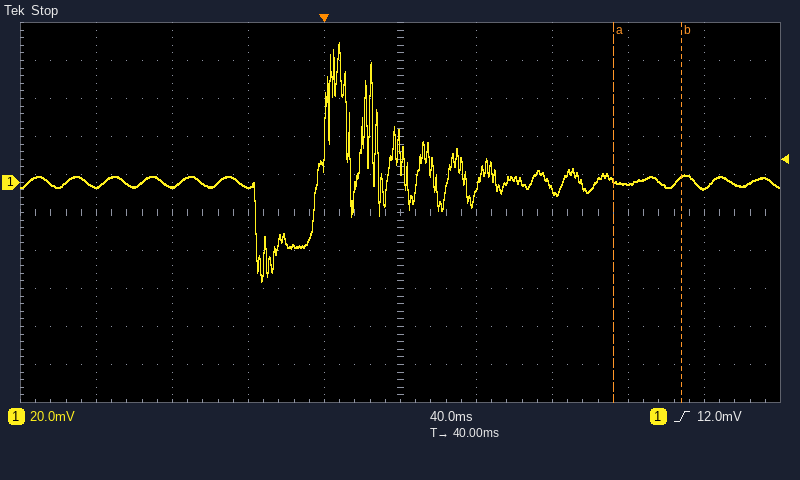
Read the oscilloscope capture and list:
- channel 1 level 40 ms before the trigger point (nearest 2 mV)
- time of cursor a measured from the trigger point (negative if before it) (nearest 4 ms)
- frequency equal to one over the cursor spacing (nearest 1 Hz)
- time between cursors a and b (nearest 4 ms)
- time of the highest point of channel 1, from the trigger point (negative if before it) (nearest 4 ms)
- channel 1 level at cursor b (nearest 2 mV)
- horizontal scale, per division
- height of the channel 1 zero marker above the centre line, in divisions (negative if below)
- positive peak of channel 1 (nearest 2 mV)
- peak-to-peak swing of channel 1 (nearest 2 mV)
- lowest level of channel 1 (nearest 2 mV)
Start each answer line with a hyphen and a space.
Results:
- -2 mV
- +152 ms
- 28 Hz
- 36 ms
- +8 ms
- 2 mV
- 40 ms
- +0.8 div
- 74 mV
- 126 mV
- -52 mV
